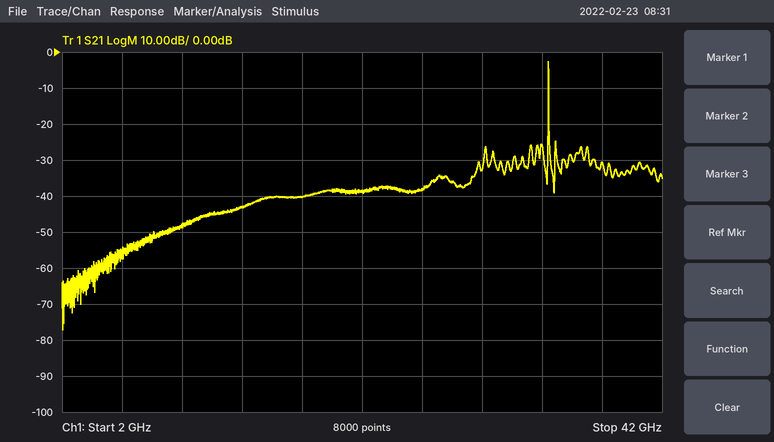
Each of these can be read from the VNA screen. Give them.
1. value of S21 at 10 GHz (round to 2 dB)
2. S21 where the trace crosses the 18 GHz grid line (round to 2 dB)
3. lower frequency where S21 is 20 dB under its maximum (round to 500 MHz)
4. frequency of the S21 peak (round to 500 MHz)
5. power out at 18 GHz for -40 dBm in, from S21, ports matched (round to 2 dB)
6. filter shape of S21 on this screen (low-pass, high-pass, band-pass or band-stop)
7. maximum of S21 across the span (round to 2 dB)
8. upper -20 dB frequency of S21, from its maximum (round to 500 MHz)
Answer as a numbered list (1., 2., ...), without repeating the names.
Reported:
1. -48 dB
2. -40 dB
3. 34.5 GHz
4. 34.5 GHz
5. -80 dBm
6. band-pass
7. -2 dB
8. 34.5 GHz
